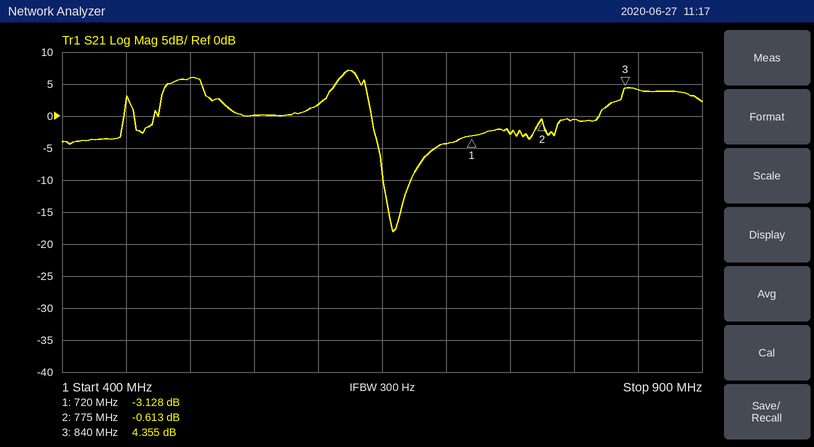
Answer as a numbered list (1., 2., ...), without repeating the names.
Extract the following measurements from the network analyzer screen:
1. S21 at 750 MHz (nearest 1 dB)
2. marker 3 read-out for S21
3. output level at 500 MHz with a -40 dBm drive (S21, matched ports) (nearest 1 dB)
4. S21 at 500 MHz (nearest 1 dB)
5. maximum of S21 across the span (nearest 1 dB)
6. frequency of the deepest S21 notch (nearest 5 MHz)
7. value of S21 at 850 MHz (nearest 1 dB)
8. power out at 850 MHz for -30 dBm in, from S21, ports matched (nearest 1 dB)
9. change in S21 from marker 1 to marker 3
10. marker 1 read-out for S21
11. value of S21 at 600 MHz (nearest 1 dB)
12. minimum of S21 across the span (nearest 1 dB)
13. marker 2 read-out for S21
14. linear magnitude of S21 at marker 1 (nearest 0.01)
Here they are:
1. -3 dB
2. 4.355 dB
3. -34 dBm
4. 6 dB
5. 7 dB
6. 660 MHz
7. 4 dB
8. -26 dBm
9. 7.483 dB
10. -3.128 dB
11. 2 dB
12. -18 dB
13. -0.613 dB
14. 0.70
